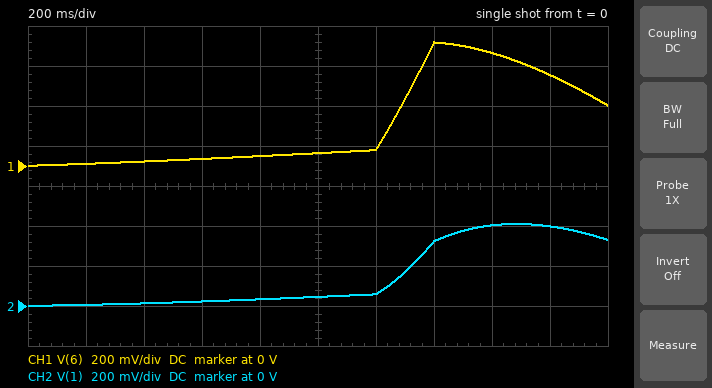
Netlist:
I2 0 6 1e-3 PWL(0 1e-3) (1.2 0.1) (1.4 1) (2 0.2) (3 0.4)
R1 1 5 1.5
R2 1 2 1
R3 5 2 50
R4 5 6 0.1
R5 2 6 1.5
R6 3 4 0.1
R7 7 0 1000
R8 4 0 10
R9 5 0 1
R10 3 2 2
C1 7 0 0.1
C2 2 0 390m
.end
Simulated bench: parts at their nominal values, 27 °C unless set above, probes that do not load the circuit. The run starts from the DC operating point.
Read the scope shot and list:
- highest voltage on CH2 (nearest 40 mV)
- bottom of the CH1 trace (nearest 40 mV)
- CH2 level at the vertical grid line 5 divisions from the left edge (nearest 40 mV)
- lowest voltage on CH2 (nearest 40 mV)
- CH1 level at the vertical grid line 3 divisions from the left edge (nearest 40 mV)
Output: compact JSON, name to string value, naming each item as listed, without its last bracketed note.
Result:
{"highest voltage on CH2": "400 mV", "bottom of the CH1 trace": "0 V", "CH2 level at the vertical grid line 5 divisions from the left edge": "40 mV", "lowest voltage on CH2": "0 V", "CH1 level at the vertical grid line 3 divisions from the left edge": "40 mV"}
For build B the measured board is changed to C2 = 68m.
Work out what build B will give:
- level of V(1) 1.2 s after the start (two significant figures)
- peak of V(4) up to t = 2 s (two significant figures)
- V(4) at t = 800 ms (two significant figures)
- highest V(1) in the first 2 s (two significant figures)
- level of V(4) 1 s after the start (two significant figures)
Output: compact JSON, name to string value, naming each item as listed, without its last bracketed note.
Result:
{"level of V(1) 1.2 s after the start": "85 mV", "peak of V(4) up to t = 2 s": "600 mV", "V(4) at t = 800 ms": "43 mV", "highest V(1) in the first 2 s": "730 mV", "level of V(4) 1 s after the start": "56 mV"}
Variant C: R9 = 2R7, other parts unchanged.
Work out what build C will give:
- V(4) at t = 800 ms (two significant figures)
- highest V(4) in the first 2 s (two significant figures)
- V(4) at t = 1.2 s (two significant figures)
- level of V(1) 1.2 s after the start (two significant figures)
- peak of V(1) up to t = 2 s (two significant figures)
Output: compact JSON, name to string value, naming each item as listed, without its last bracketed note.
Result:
{"V(4) at t = 800 ms": "35 mV", "highest V(4) in the first 2 s": "550 mV", "V(4) at t = 1.2 s": "70 mV", "level of V(1) 1.2 s after the start": "100 mV", "peak of V(1) up to t = 2 s": "710 mV"}
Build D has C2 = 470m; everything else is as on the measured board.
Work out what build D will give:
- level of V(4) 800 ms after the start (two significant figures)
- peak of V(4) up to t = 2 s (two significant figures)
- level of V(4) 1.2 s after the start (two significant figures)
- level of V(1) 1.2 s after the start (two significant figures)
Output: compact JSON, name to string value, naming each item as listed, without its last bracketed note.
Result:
{"level of V(4) 800 ms after the start": "19 mV", "peak of V(4) up to t = 2 s": "290 mV", "level of V(4) 1.2 s after the start": "37 mV", "level of V(1) 1.2 s after the start": "54 mV"}
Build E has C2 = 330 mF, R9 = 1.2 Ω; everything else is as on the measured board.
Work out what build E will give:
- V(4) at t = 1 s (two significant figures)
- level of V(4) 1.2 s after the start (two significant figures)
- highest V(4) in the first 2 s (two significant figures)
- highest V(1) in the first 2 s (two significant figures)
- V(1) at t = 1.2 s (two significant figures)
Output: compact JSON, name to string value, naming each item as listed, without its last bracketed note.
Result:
{"V(4) at t = 1 s": "38 mV", "level of V(4) 1.2 s after the start": "50 mV", "highest V(4) in the first 2 s": "390 mV", "highest V(1) in the first 2 s": "500 mV", "V(1) at t = 1.2 s": "70 mV"}
